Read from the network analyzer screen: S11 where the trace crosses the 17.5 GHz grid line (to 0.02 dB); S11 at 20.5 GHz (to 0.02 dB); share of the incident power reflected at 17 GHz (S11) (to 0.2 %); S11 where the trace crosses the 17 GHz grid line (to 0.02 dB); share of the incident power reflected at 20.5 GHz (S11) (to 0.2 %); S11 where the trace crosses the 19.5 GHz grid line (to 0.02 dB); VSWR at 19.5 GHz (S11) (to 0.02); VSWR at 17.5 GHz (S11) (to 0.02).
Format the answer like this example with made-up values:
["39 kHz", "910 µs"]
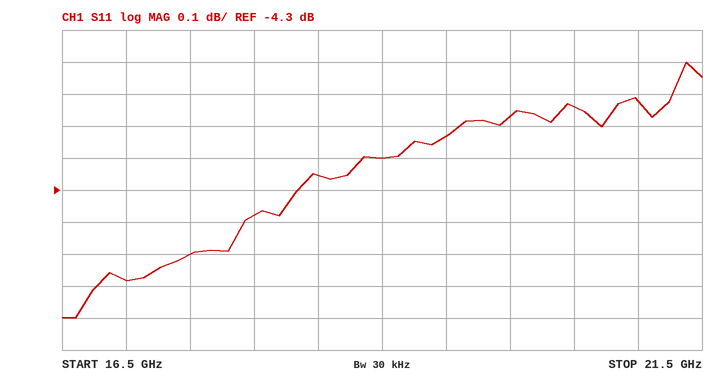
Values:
["-4.50 dB", "-4.04 dB", "34.8 %", "-4.58 dB", "39.4 %", "-4.14 dB", "4.28", "3.94"]
